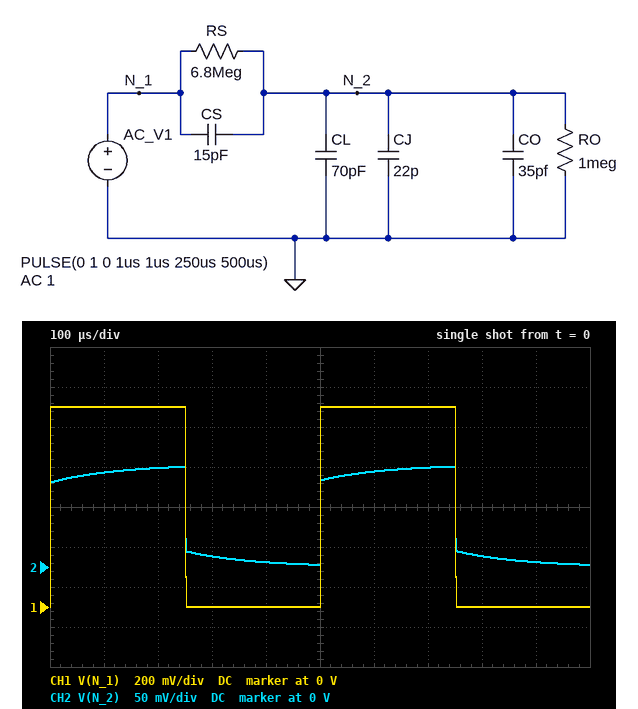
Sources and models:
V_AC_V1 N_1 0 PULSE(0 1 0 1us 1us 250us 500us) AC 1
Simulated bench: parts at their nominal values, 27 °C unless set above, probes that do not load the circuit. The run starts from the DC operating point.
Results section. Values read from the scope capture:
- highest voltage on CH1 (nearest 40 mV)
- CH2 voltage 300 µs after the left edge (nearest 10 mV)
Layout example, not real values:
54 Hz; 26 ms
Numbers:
1.00 V; 10 mV
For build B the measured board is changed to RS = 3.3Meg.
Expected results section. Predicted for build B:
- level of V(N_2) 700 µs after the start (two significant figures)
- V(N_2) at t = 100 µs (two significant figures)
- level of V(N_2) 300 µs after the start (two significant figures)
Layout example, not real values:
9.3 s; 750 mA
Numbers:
210 mV; 180 mV; 73 mV
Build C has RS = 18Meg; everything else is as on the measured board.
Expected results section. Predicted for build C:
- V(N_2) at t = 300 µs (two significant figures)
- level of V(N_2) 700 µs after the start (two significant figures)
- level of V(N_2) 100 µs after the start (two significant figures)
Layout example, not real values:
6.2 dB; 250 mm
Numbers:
-31 mV; 63 mV; 78 mV
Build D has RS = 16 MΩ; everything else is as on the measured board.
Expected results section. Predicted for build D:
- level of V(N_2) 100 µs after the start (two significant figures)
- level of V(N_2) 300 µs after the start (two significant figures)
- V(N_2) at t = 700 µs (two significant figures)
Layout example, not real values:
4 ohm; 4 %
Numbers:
81 mV; -28 mV; 68 mV
